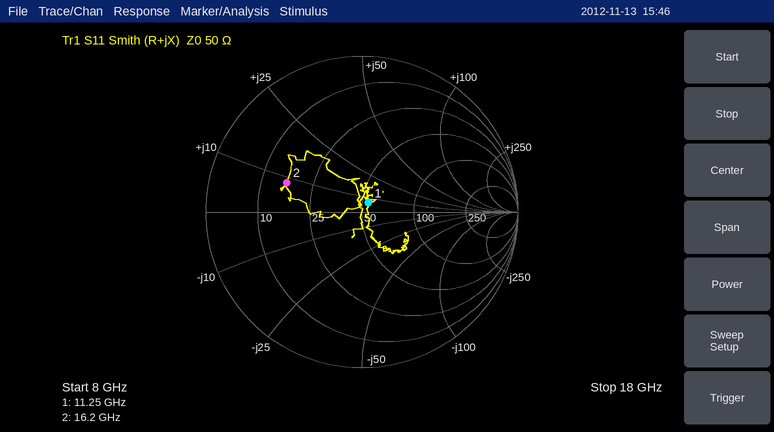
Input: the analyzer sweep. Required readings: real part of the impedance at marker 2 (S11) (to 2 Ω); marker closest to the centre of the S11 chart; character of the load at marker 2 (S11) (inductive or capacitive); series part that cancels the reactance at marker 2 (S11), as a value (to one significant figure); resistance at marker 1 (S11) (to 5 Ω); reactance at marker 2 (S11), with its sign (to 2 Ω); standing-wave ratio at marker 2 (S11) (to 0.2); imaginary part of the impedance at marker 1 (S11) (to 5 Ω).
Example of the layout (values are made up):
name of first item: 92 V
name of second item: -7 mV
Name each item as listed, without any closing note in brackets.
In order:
real part of the impedance at marker 2 (S11): 16 Ω
marker closest to the centre of the S11 chart: marker 1
character of the load at marker 2 (S11): inductive
series part that cancels the reactance at marker 2 (S11), as a value: 1 pF
resistance at marker 1 (S11): 55 Ω
reactance at marker 2 (S11), with its sign: +8 Ω
standing-wave ratio at marker 2 (S11): 3.2
imaginary part of the impedance at marker 1 (S11): +5 Ω
